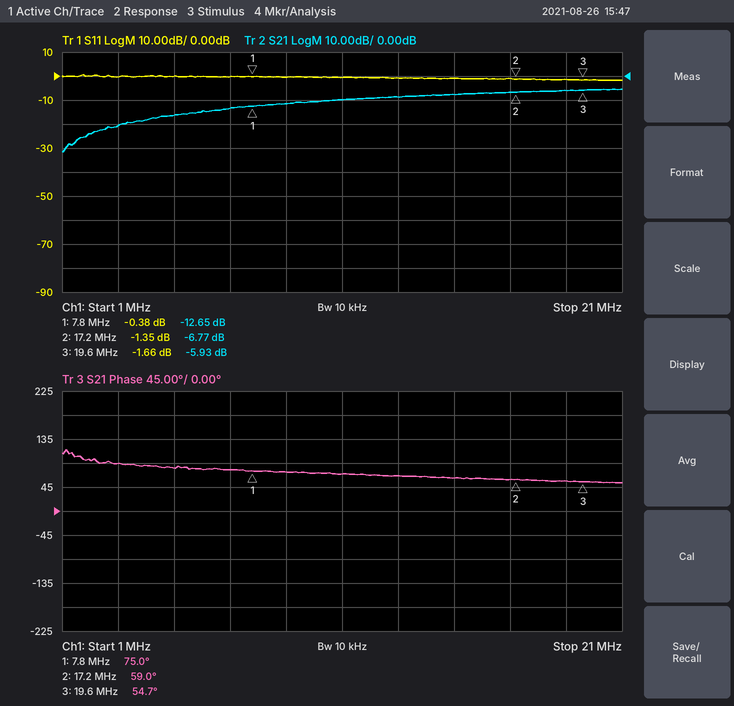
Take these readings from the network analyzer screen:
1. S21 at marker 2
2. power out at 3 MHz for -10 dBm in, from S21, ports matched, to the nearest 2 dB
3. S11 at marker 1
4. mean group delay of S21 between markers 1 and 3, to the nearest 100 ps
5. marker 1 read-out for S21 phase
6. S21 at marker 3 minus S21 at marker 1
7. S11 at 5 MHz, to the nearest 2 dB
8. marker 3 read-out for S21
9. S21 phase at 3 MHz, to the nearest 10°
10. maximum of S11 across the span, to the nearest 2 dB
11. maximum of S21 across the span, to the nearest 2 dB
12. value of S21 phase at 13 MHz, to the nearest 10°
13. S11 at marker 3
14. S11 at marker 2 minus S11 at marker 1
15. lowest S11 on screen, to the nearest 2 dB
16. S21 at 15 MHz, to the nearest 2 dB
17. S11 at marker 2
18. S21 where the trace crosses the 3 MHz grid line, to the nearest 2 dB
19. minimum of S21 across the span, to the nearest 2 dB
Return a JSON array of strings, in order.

["-6.77 dB", "-30 dBm", "-0.38 dB", "4.8 ns", "75.0°", "6.72 dB", "0 dB", "-5.93 dB", "90°", "0 dB", "-6 dB", "70°", "-1.66 dB", "-0.97 dB", "-2 dB", "-8 dB", "-1.35 dB", "-20 dB", "-32 dB"]
